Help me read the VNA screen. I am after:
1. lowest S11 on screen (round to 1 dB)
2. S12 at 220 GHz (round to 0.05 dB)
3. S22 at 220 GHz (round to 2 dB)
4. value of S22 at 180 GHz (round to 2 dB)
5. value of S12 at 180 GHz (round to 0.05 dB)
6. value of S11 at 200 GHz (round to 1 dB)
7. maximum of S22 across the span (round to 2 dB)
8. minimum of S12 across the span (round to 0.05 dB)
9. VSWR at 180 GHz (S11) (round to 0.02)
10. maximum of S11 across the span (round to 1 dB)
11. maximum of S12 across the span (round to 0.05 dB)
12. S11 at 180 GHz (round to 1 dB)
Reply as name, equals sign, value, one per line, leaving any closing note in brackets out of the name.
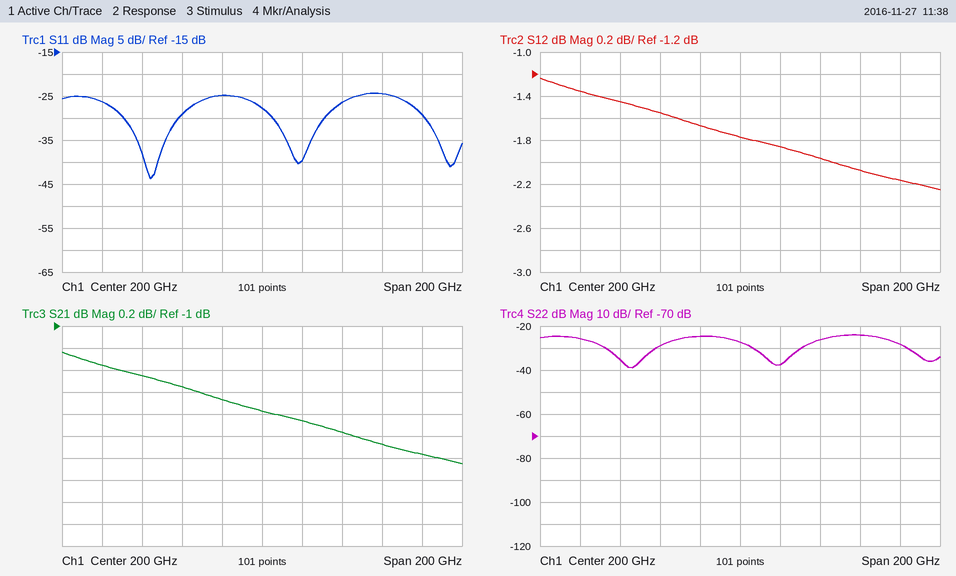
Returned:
lowest S11 on screen = -44 dB
S12 at 220 GHz = -1.85 dB
S22 at 220 GHz = -38 dB
value of S22 at 180 GHz = -24 dB
value of S12 at 180 GHz = -1.65 dB
value of S11 at 200 GHz = -28 dB
maximum of S22 across the span = -24 dB
minimum of S12 across the span = -2.25 dB
VSWR at 180 GHz (S11) = 1.12
maximum of S11 across the span = -24 dB
maximum of S12 across the span = -1.25 dB
S11 at 180 GHz = -25 dB
